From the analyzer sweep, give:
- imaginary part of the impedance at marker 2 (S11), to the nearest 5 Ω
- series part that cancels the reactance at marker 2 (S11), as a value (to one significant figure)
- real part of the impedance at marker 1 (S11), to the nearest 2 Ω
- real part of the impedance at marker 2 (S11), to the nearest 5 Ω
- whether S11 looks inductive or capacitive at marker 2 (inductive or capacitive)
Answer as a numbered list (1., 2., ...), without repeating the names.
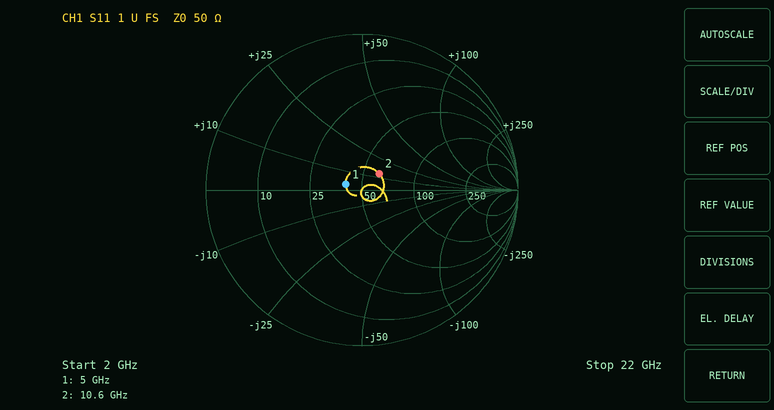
1. +15 Ω
2. 1 pF
3. 40 Ω
4. 60 Ω
5. inductive
